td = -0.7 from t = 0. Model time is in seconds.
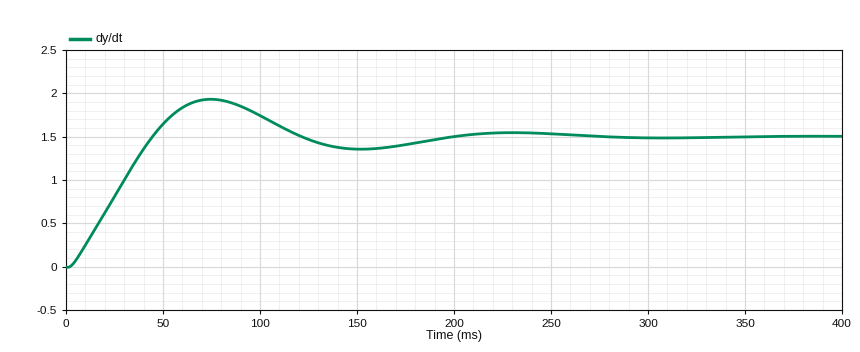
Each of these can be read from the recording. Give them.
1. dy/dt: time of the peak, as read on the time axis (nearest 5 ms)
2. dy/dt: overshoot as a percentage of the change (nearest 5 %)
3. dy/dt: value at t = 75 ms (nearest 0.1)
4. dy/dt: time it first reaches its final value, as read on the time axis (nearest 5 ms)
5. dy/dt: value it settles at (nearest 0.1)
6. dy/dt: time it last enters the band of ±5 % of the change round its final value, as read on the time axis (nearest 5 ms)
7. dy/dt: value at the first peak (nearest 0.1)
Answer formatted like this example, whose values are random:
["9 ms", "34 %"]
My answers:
["75 ms", "30 %", "1.9", "45 ms", "1.5", "180 ms", "1.9"]
